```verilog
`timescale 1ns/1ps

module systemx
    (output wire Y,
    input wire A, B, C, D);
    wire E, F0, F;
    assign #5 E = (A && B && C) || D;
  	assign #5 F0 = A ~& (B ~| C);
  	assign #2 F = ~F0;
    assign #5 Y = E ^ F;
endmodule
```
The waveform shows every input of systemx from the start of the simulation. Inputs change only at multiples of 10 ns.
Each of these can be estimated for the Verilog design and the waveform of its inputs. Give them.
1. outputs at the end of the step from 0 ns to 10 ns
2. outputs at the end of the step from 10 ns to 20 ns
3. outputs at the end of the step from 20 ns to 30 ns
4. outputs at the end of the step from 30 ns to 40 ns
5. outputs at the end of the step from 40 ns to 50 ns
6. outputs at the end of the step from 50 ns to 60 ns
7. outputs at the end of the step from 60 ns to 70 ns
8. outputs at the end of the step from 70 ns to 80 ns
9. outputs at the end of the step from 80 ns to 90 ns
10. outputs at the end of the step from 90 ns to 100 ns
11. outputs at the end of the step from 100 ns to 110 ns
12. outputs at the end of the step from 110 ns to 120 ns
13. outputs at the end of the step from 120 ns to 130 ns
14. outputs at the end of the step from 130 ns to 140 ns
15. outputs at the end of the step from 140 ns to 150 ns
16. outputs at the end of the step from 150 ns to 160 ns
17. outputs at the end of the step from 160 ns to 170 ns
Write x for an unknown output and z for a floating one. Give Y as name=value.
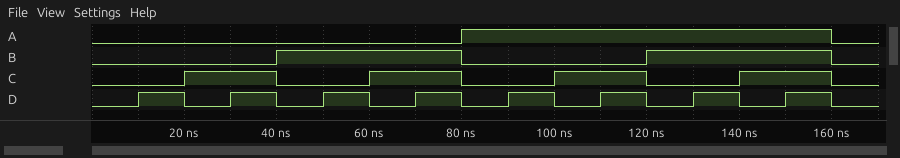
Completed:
Y=x
Y=0
Y=1
Y=0
Y=1
Y=0
Y=1
Y=0
Y=1
Y=1
Y=0
Y=0
Y=1
Y=0
Y=1
Y=1
Y=1
